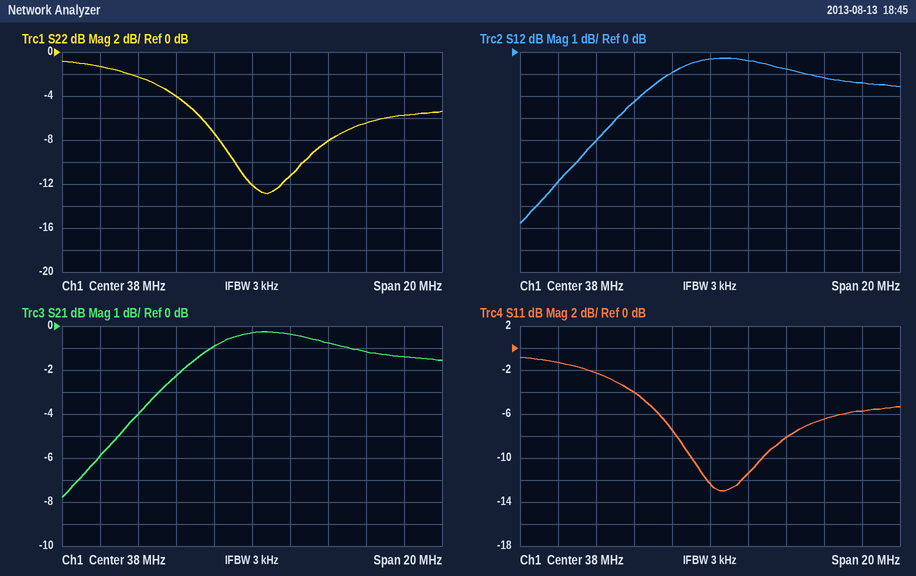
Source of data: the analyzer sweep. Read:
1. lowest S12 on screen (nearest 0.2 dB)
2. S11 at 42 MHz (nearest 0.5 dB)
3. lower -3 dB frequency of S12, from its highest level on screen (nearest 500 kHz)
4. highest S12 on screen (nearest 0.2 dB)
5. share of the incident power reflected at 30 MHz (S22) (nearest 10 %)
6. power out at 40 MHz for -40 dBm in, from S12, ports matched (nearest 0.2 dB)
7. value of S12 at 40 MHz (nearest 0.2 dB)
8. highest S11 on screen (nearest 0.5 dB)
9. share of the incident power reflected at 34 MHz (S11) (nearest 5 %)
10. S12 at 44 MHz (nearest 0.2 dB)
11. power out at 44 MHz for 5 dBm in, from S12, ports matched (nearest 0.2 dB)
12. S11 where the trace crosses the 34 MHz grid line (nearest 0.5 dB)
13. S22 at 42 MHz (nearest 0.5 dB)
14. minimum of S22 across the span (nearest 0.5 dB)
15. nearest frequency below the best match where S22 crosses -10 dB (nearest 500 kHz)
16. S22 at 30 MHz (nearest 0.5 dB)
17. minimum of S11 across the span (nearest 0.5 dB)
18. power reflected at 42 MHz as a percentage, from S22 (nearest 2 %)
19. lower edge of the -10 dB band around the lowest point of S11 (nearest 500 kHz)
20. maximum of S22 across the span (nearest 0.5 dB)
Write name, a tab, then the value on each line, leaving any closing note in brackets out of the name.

lowest S12 on screen	-7.8 dB
S11 at 42 MHz	-8.0 dB
lower -3 dB frequency of S12, from its highest level on screen	33.0 MHz
highest S12 on screen	-0.2 dB
share of the incident power reflected at 30 MHz (S22)	70 %
power out at 40 MHz for -40 dBm in, from S12, ports matched	-40.4 dBm
value of S12 at 40 MHz	-0.4 dB
highest S11 on screen	-1.0 dB
share of the incident power reflected at 34 MHz (S11)	40 %
S12 at 44 MHz	-1.2 dB
power out at 44 MHz for 5 dBm in, from S12, ports matched	3.8 dBm
S11 where the trace crosses the 34 MHz grid line	-4.0 dB
S22 at 42 MHz	-8.0 dB
minimum of S22 across the span	-13.0 dB
nearest frequency below the best match where S22 crosses -10 dB	37.0 MHz
S22 at 30 MHz	-1.5 dB
minimum of S11 across the span	-13.0 dB
power reflected at 42 MHz as a percentage, from S22	16 %
lower edge of the -10 dB band around the lowest point of S11	37.0 MHz
maximum of S22 across the span	-1.0 dB
